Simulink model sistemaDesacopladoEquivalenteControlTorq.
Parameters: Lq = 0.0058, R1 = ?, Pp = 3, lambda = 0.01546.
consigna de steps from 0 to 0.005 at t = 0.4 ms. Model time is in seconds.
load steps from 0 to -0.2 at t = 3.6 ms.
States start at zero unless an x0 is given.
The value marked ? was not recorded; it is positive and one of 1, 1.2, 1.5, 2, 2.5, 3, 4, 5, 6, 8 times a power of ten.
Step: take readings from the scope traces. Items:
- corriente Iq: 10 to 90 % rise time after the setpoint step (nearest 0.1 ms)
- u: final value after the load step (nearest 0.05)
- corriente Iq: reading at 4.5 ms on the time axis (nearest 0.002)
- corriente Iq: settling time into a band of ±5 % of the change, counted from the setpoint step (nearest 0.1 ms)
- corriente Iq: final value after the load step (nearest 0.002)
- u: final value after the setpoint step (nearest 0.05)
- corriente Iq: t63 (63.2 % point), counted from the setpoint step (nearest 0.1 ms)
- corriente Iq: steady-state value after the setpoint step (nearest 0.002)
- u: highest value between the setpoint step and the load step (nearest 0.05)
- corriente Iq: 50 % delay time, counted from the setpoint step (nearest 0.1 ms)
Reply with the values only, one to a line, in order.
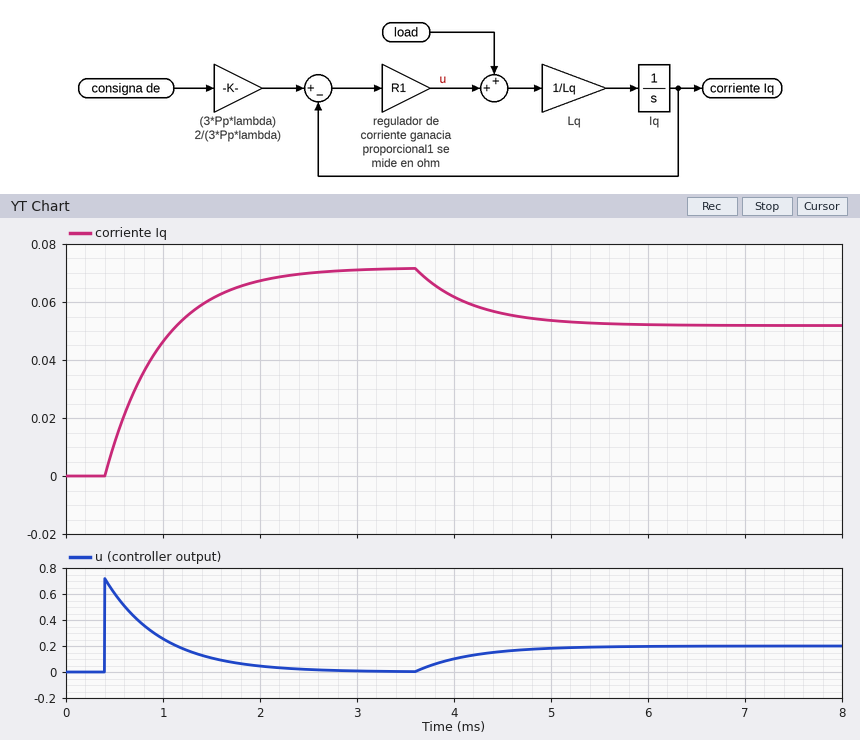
1.3 ms
0.20
0.056
1.7 ms
0.052
0.00
0.6 ms
0.072
0.70
0.4 ms
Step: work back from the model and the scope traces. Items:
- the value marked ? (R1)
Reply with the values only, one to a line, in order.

10
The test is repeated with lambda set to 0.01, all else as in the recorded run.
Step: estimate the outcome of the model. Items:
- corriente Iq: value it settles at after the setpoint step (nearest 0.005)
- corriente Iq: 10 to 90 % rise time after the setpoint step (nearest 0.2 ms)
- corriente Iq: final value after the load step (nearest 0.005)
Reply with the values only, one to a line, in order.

0.110
1.2 ms
0.090
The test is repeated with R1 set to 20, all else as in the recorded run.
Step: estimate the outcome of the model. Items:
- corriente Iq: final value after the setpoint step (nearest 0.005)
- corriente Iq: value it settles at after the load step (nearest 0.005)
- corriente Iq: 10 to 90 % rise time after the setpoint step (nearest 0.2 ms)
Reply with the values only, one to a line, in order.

0.070
0.060
0.6 ms
